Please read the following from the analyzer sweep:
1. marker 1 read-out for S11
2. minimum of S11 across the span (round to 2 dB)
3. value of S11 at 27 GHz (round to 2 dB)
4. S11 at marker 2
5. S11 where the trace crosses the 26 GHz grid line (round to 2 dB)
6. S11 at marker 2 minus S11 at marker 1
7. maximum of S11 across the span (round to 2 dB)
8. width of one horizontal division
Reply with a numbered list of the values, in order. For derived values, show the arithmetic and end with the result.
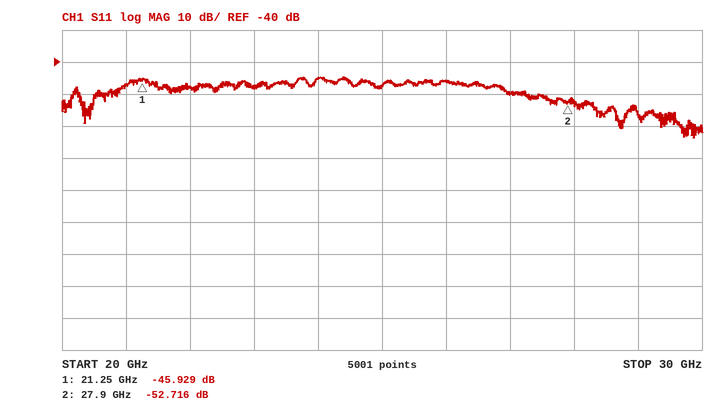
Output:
1. -45.929 dB
2. -64 dB
3. -50 dB
4. -52.716 dB
5. -46 dB
6. -52.716 − (-45.929) = -6.787 dB
7. -44 dB
8. 1 GHz
